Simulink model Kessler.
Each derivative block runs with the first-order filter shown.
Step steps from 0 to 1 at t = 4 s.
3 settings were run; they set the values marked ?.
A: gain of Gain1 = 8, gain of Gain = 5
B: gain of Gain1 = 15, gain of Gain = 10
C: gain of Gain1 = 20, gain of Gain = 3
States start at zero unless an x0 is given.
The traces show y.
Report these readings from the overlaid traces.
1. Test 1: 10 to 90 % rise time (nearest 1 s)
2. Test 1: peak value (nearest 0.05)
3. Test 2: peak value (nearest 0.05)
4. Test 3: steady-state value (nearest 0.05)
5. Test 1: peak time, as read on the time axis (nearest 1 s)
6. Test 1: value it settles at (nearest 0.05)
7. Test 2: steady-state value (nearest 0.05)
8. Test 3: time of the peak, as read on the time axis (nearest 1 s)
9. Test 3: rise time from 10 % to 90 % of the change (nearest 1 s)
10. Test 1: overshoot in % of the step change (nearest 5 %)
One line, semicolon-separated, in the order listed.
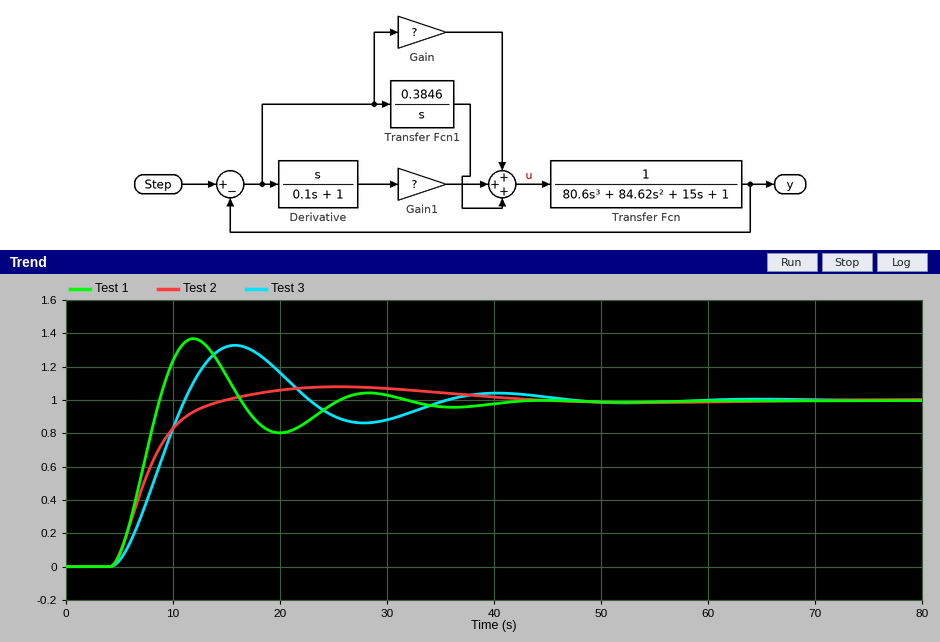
3 s; 1.35; 1.10; 1.00; 12 s; 1.00; 1.00; 16 s; 5 s; 35 %
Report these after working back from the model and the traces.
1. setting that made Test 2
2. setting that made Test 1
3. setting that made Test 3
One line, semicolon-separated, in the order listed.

C; B; A
